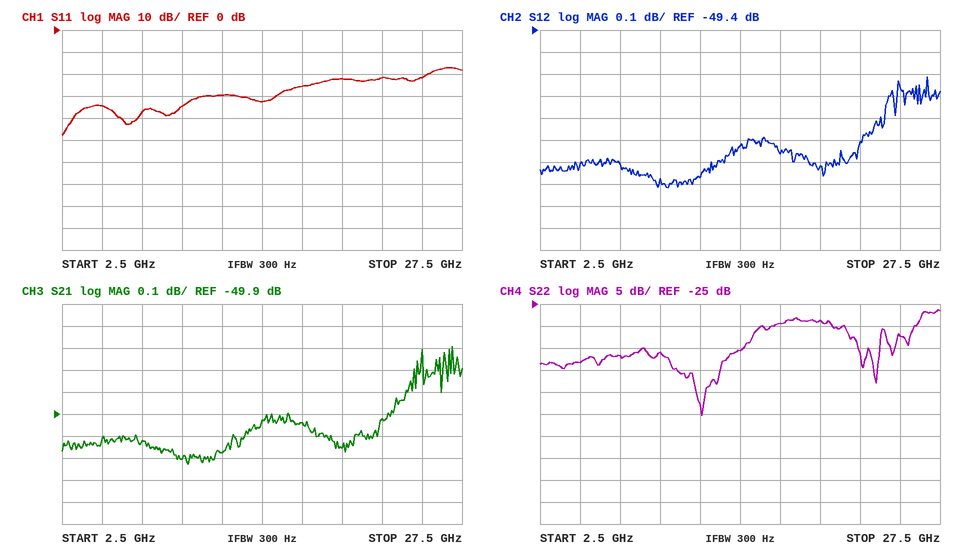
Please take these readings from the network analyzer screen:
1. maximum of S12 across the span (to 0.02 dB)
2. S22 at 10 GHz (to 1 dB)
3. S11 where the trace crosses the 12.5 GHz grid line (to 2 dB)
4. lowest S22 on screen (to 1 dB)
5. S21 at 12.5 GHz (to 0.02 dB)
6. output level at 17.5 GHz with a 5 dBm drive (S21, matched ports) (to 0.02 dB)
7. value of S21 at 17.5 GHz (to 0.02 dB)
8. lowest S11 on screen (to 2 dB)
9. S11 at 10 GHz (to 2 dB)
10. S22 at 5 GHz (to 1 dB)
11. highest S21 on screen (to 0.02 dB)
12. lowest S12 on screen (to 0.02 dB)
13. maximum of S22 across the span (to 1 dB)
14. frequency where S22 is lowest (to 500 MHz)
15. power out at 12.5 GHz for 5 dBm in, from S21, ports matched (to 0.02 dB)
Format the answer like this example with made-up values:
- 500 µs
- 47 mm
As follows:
- -49.62 dB
- -36 dB
- -30 dB
- -50 dB
- -50.08 dB
- -44.94 dBm
- -49.94 dB
- -48 dB
- -34 dB
- -38 dB
- -49.60 dB
- -50.12 dB
- -26 dB
- 12.5 GHz
- -45.08 dBm
